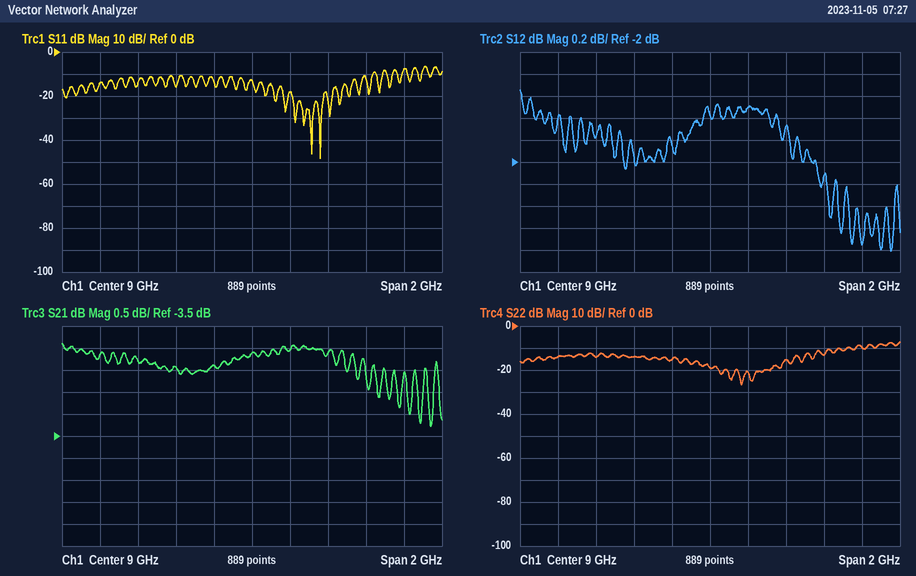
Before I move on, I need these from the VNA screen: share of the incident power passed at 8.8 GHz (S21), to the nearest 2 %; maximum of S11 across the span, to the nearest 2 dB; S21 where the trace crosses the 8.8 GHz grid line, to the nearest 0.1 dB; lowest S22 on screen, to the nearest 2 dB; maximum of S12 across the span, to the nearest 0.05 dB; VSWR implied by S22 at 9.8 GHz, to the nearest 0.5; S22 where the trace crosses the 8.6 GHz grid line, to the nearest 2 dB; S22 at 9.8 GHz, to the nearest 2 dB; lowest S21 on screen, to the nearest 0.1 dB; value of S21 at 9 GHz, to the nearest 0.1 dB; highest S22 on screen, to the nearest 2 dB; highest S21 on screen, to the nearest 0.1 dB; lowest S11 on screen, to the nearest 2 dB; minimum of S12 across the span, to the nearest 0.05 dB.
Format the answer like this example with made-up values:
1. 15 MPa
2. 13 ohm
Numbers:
1. 64 %
2. -6 dB
3. -1.9 dB
4. -26 dB
5. -1.35 dB
6. 2.0
7. -14 dB
8. -10 dB
9. -3.3 dB
10. -1.6 dB
11. -8 dB
12. -1.4 dB
13. -48 dB
14. -2.80 dB
